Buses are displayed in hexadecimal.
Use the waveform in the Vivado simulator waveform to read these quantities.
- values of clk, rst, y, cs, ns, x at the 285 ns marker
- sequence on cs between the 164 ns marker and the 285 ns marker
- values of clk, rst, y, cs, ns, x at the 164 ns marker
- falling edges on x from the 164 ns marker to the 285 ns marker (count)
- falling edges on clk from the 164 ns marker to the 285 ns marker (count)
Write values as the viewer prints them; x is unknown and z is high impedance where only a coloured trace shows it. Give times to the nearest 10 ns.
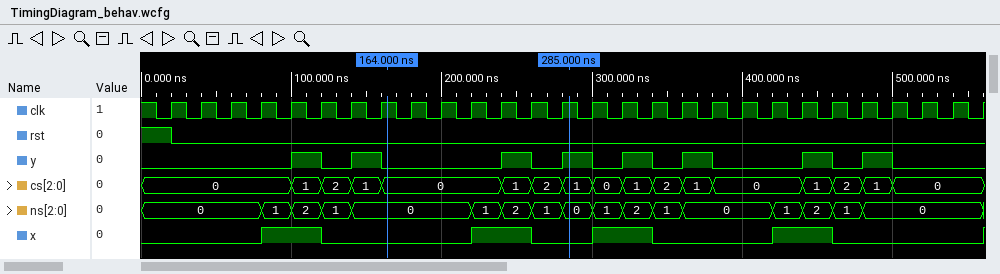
clk=1, rst=0, y=1, cs=1, ns=0, x=0
0, 1, 2, 1
clk=1, rst=0, y=0, cs=0, ns=0, x=0
1
6
